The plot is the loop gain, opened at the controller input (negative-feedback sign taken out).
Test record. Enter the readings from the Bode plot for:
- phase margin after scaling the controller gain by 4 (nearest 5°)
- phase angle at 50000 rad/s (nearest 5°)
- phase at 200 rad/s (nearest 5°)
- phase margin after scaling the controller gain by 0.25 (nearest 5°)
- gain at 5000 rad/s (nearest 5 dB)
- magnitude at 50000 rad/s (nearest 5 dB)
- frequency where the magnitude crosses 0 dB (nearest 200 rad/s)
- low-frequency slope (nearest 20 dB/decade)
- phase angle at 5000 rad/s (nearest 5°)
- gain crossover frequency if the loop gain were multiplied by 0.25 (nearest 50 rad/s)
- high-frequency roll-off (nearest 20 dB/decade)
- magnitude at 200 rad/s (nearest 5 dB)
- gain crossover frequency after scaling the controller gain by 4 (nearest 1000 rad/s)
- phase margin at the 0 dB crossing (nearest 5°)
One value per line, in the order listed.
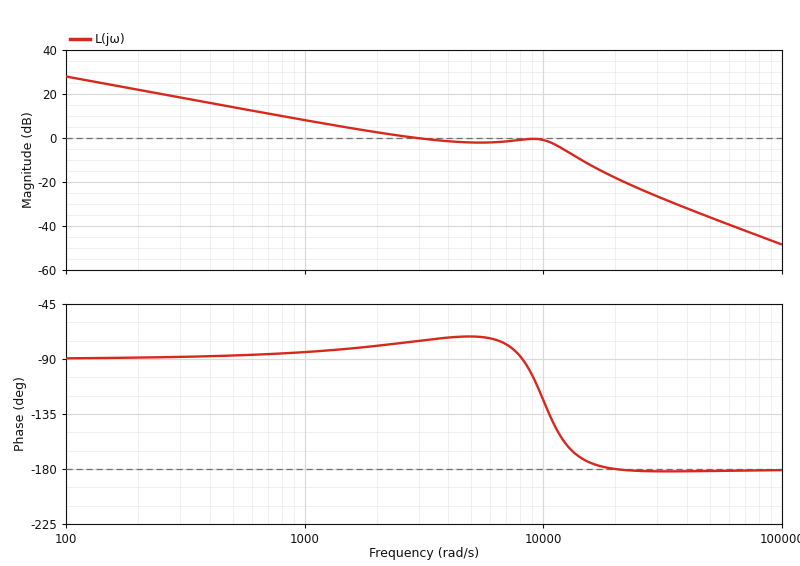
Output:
5°
-180°
-90°
95°
0 dB
-35 dB
3000 rad/s
-20 dB/decade
-70°
650 rad/s
-40 dB/decade
20 dB
16000 rad/s
105°
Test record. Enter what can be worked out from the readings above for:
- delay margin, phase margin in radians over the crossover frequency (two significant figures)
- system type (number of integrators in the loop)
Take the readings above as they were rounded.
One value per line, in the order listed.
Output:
0.00061 s
1
